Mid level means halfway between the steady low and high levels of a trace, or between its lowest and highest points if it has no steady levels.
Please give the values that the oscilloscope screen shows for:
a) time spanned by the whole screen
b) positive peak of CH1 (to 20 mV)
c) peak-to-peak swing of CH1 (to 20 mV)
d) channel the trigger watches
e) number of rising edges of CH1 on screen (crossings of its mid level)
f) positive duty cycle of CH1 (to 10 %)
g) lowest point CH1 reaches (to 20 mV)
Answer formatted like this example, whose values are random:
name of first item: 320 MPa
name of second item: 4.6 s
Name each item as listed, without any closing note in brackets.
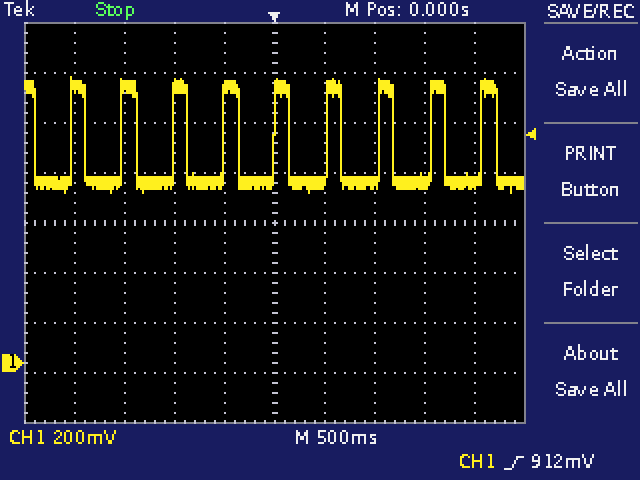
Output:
time spanned by the whole screen: 5 s
positive peak of CH1: 1.14 V
peak-to-peak swing of CH1: 460 mV
channel the trigger watches: CH1
number of rising edges of CH1 on screen: 9
positive duty cycle of CH1: 30 %
lowest point CH1 reaches: 680 mV
